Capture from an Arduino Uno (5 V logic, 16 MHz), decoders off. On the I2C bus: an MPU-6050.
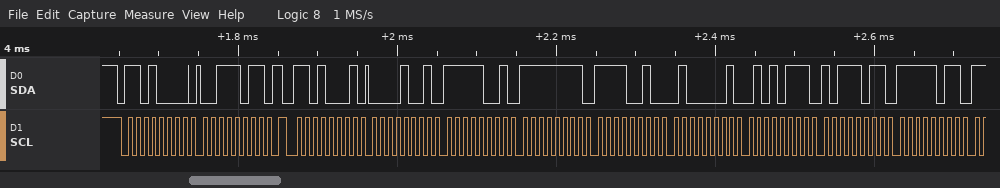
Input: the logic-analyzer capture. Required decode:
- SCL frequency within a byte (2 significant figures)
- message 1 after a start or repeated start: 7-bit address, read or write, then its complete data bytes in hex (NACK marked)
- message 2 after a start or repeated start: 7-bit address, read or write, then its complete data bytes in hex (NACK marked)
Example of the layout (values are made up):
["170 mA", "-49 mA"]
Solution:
["100 kHz", "0x68 write: 3B", "0x68 read: 09 F9 FF F2 41 57 BB FB"]
